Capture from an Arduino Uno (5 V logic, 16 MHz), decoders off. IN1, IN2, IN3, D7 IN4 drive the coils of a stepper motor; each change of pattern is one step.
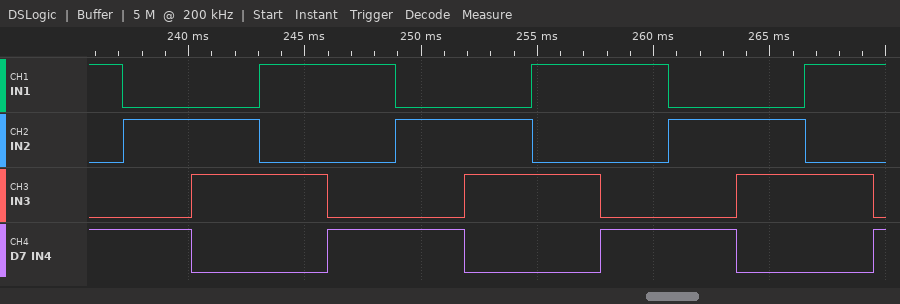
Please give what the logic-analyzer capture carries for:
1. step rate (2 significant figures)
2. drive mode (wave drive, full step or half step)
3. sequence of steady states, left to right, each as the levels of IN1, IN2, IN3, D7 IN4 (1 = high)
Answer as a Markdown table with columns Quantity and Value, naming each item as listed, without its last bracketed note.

| Quantity | Value |
|---|---|
| step rate | 340 steps/s |
| drive mode | full step |
| sequence of steady states, left to right, each as the levels of IN1, IN2, IN3, D7 IN4 | 1001 0101 0110 1010 1001 0101 0110 1010 1001 0101 0110 1010 1001 |
